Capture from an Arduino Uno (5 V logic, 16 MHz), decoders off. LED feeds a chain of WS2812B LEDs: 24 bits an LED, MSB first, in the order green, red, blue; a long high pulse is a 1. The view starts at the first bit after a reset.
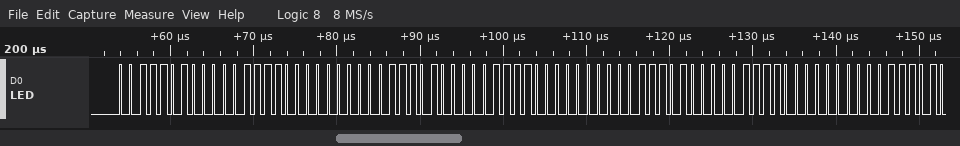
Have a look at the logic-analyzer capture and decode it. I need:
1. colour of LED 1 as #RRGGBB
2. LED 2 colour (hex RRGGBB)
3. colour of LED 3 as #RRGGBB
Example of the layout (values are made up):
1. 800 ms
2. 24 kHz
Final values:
1. #0F3A00
2. #0F3A00
3. #0F3A00
